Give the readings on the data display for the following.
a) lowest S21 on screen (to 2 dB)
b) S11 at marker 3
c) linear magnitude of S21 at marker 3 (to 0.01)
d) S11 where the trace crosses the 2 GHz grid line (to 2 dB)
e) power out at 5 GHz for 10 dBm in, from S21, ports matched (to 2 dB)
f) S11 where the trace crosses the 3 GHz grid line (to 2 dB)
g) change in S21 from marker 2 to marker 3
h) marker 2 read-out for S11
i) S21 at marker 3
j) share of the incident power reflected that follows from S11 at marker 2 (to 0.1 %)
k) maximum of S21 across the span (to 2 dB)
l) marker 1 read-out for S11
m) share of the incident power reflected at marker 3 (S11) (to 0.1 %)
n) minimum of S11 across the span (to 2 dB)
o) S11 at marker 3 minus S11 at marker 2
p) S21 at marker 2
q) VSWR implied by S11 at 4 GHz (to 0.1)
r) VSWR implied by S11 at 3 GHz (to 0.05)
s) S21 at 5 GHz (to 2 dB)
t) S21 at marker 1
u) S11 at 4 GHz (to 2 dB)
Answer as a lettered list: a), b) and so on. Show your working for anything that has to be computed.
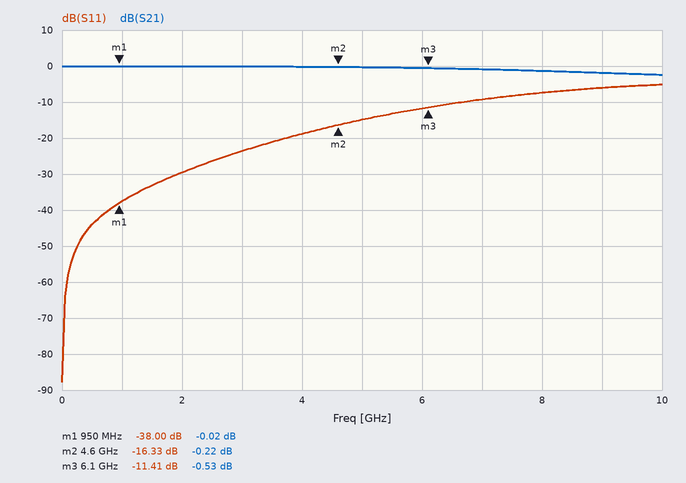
a) -2 dB
b) -11.41 dB
c) 10^(-0.53/20) ≈ 0.94
d) -30 dB
e) 10 dBm + (0 dB) = 10 dBm
f) -24 dB
g) -0.53 − (-0.22) = -0.31 dB
h) -16.33 dB
i) -0.53 dB
j) 10^(-16.33/10) ≈ 2.3 %
k) 0 dB
l) -38.00 dB
m) 10^(-11.41/10) ≈ 7.2 %
n) -88 dB
o) -11.41 − (-16.33) = 4.92 dB
p) -0.22 dB
q) |Γ| = 10^(-18/20) = 0.1259; VSWR = (1 + 0.1259)/(1 − 0.1259) ≈ 1.3
r) |Γ| = 10^(-24/20) = 0.0631; VSWR = (1 + 0.0631)/(1 − 0.0631) ≈ 1.13, so 1.15 to the nearest 0.05
s) 0 dB
t) -0.02 dB
u) -18 dB
